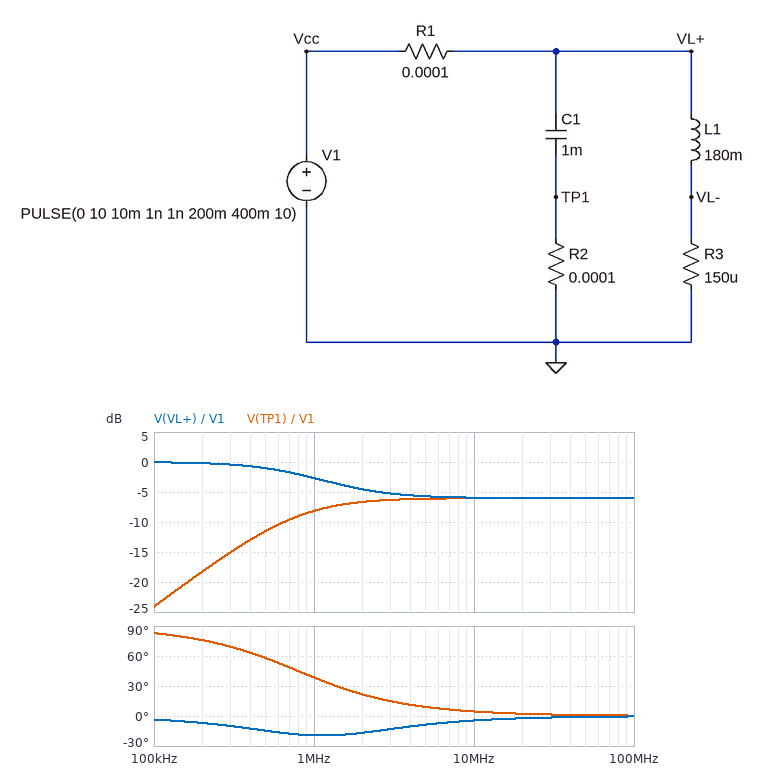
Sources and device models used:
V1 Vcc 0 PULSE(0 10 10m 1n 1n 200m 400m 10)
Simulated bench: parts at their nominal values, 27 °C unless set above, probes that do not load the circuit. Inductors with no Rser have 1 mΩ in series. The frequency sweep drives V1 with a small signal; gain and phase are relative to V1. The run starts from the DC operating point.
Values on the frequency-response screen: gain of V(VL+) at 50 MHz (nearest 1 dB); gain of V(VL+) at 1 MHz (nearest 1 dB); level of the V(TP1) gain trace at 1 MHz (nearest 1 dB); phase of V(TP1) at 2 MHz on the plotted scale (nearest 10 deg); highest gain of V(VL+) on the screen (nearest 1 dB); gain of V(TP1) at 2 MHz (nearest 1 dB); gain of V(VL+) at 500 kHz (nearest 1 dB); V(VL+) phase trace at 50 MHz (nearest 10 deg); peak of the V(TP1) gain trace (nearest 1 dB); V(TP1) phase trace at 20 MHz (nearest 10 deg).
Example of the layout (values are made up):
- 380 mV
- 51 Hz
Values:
- -6 dB
- -3 dB
- -8 dB
- 20 deg
- 0 dB
- -7 dB
- -1 dB
- 0 deg
- -6 dB
- 0 deg
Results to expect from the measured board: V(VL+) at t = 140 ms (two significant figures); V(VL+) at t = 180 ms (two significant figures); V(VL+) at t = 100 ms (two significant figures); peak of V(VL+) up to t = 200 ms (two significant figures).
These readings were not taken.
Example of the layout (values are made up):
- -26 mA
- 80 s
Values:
- 10 V
- 10 V
- 10 V
- 10 V
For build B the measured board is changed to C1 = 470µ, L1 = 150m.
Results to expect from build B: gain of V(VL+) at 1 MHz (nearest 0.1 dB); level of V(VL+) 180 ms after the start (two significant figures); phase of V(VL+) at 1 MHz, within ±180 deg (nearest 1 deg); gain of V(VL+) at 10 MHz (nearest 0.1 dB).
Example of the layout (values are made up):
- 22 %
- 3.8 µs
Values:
- -0.9 dB
- 10 V
- -14 deg
- -5.7 dB
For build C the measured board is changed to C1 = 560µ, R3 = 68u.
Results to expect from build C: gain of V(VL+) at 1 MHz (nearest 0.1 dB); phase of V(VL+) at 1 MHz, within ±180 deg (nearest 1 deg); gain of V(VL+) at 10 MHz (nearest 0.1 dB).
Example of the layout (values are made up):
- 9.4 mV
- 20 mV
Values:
- -1.2 dB
- -16 deg
- -5.8 dB
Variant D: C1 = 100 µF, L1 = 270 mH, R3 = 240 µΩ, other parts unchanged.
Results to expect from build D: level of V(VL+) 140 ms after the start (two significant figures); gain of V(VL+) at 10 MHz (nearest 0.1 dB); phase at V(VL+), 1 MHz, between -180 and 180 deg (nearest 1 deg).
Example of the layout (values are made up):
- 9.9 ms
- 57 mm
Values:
- 10 V
- -2.7 dB
- -4 deg
